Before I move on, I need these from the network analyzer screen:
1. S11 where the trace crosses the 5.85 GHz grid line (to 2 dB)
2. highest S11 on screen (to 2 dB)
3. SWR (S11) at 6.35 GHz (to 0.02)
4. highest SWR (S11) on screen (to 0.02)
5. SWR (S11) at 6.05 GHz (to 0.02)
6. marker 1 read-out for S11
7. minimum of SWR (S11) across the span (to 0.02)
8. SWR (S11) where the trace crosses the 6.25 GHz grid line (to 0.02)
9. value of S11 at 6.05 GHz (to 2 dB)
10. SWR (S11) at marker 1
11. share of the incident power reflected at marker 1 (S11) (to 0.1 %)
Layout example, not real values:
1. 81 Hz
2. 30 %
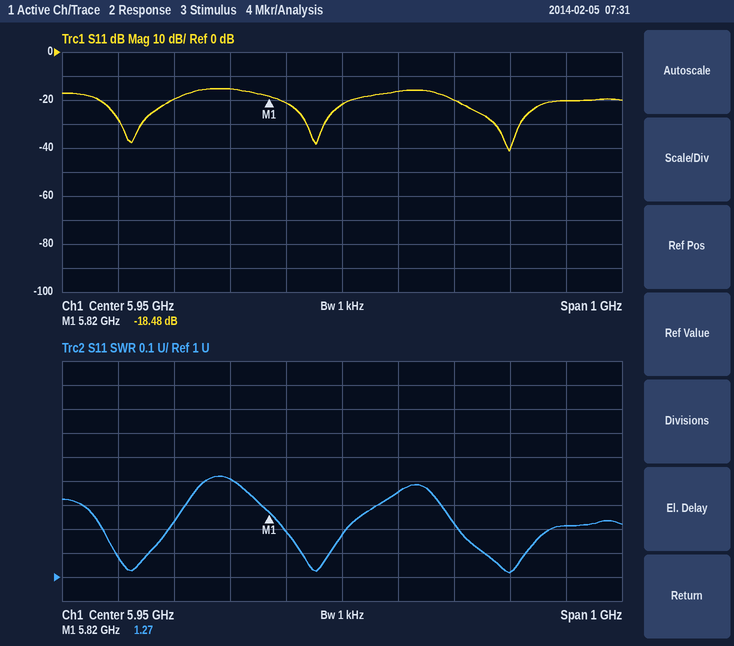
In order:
1. -22 dB
2. -16 dB
3. 1.22
4. 1.42
5. 1.36
6. -18.48 dB
7. 1.02
8. 1.02
9. -16 dB
10. 1.27
11. 1.4 %
